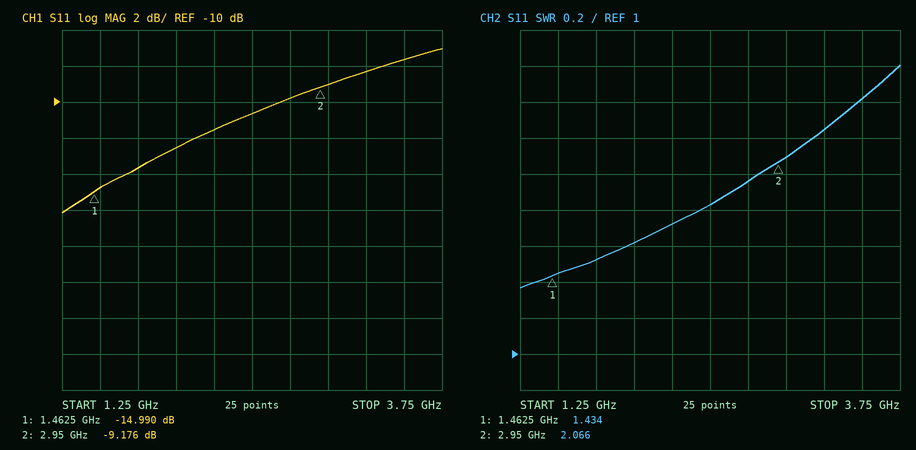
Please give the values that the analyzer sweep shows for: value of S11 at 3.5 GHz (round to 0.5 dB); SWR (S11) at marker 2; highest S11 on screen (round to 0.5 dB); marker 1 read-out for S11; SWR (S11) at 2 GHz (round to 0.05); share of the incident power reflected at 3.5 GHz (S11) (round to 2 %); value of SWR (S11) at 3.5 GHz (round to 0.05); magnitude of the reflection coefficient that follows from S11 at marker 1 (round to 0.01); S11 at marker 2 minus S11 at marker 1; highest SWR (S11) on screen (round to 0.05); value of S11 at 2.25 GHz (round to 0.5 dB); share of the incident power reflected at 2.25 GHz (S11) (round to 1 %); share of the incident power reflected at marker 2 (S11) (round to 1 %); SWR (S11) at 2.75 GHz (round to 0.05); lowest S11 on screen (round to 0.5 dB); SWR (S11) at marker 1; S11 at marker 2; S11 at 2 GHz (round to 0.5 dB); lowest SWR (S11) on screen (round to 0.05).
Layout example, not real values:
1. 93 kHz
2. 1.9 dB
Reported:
1. -7.5 dB
2. 2.066
3. -7.0 dB
4. -14.990 dB
5. 1.60
6. 18 %
7. 2.40
8. 0.18
9. 5.814 dB
10. 2.60
11. -11.5 dB
12. 7 %
13. 12 %
14. 1.95
15. -16.0 dB
16. 1.434
17. -9.176 dB
18. -12.5 dB
19. 1.35
